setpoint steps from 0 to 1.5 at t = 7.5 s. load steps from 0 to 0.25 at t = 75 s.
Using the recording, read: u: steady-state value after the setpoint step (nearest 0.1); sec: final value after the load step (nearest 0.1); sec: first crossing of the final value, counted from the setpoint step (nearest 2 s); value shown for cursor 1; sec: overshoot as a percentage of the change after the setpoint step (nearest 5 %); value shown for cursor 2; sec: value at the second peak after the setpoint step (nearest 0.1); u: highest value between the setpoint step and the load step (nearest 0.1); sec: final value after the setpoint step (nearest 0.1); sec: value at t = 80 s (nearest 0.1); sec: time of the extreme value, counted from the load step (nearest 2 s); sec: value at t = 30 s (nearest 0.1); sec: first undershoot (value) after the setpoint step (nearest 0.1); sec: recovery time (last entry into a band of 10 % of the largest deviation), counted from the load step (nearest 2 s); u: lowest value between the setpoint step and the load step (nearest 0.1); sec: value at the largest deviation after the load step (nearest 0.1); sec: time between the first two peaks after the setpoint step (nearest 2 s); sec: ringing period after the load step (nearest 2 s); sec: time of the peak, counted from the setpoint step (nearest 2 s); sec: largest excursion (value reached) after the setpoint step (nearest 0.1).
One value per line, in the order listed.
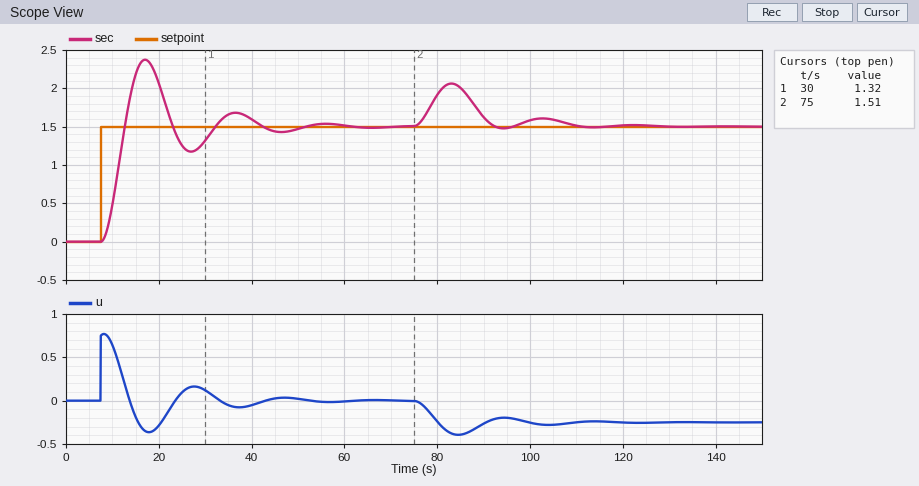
0.0
1.5
6 s
1.32
60 %
1.51
1.7
0.8
1.5
1.9
8 s
1.3
1.2
32 s
-0.4
2.1
20 s
20 s
10 s
2.4
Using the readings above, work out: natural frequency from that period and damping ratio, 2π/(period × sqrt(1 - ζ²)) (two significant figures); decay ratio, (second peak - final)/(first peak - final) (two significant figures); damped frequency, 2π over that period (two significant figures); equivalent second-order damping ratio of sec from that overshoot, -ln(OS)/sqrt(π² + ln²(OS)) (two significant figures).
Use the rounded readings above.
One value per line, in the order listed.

0.32 rad/s
0.22
0.31 rad/s
0.16
